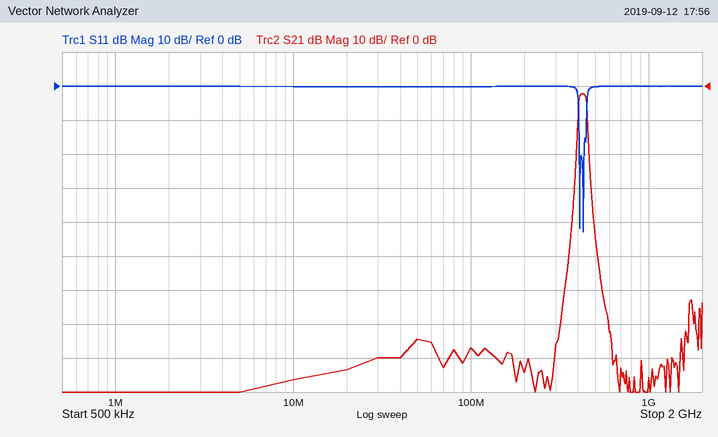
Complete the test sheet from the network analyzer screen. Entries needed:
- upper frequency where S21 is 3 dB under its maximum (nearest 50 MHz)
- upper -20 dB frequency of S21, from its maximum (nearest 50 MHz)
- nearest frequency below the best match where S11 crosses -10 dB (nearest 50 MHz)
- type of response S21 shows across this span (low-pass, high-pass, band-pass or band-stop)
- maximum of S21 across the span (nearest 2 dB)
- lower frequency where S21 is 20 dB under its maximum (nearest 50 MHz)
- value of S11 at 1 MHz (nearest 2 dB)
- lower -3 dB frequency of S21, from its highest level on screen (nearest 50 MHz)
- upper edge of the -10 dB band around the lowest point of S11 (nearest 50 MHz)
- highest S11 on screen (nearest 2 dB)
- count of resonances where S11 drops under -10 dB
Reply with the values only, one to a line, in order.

450 MHz
450 MHz
400 MHz
band-pass
-2 dB
400 MHz
0 dB
400 MHz
450 MHz
0 dB
2
